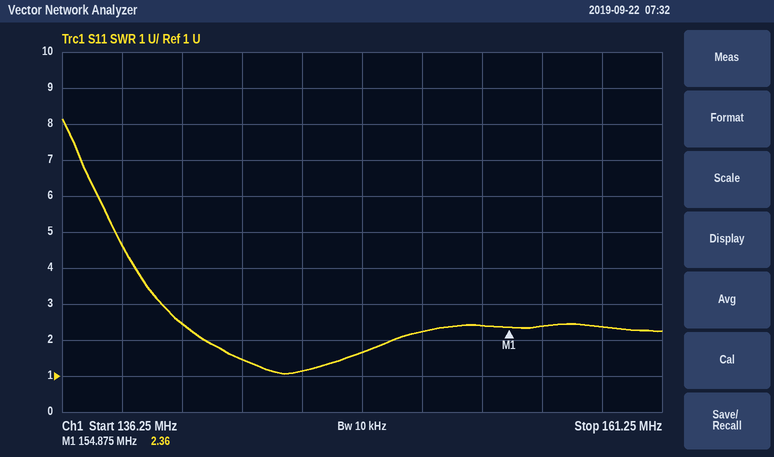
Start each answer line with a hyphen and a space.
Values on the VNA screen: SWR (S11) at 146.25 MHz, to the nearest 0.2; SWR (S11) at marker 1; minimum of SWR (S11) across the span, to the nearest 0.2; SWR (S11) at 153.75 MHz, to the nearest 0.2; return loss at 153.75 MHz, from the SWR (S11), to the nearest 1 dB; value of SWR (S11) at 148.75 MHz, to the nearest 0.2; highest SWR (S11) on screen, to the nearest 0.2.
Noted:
- 1.2
- 2.36
- 1.0
- 2.4
- 8 dB
- 1.6
- 8.2
